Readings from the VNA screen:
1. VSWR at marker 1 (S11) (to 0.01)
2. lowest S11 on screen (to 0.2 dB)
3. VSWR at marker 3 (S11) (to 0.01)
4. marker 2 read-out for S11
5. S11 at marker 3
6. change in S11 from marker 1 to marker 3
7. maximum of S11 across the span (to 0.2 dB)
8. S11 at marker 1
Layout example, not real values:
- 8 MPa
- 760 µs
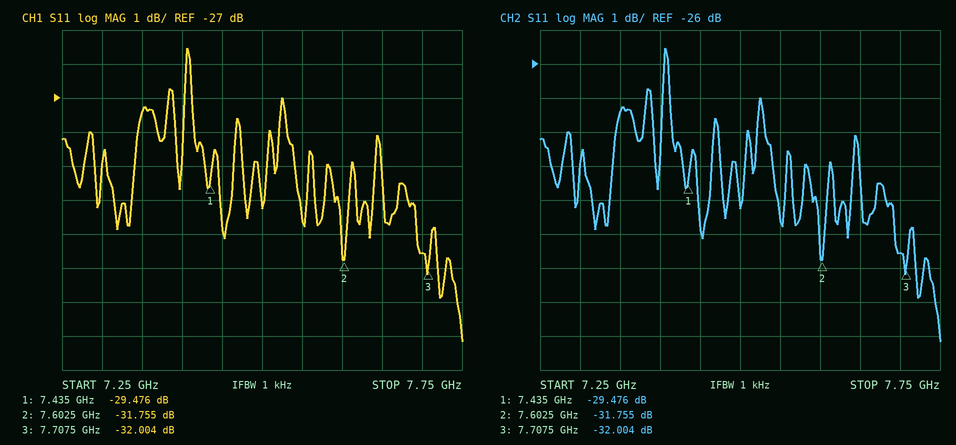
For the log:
- 1.07
- -34.2 dB
- 1.05
- -31.755 dB
- -32.004 dB
- -2.528 dB
- -25.6 dB
- -29.476 dB
